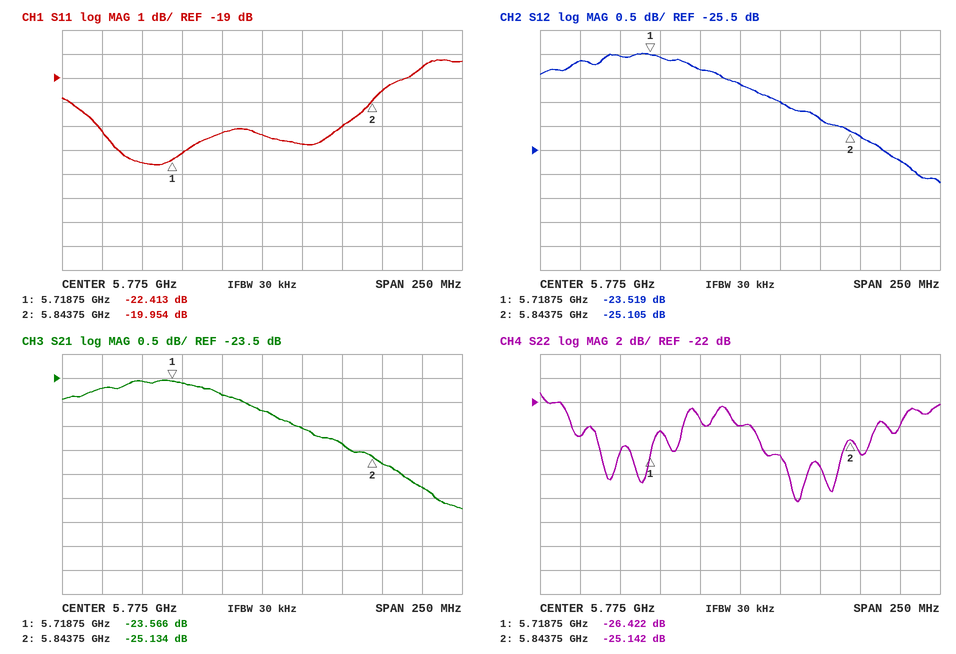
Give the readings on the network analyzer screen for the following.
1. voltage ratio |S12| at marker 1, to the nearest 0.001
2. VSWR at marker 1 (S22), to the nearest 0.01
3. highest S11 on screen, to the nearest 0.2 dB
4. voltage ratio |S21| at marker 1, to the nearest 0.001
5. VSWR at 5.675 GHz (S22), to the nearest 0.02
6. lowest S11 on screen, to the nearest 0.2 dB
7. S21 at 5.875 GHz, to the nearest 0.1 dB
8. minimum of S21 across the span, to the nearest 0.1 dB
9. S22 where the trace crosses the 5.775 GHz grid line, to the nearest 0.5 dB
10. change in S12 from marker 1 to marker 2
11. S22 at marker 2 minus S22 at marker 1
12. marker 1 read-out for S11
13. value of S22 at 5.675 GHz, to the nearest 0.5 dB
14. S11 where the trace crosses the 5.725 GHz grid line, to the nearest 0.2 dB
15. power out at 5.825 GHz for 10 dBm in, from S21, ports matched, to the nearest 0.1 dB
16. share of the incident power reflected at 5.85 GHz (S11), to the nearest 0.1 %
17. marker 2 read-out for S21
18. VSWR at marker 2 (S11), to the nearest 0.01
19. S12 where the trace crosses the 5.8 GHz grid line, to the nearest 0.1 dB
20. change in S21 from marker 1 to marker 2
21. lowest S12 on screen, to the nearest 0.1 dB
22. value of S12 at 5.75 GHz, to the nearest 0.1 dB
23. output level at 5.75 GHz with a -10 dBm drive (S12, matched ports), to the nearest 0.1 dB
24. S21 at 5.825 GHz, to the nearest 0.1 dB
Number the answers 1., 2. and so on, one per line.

1. 0.067
2. 1.10
3. -18.2 dB
4. 0.066
5. 1.12
6. -22.6 dB
7. -25.8 dB
8. -26.2 dB
9. -24.0 dB
10. -1.586 dB
11. 1.280 dB
12. -22.413 dB
13. -25.0 dB
14. -22.2 dB
15. -14.9 dBm
16. 1.1 %
17. -25.134 dB
18. 1.22
19. -24.5 dB
20. -1.568 dB
21. -26.2 dB
22. -23.8 dB
23. -33.8 dBm
24. -24.9 dB
